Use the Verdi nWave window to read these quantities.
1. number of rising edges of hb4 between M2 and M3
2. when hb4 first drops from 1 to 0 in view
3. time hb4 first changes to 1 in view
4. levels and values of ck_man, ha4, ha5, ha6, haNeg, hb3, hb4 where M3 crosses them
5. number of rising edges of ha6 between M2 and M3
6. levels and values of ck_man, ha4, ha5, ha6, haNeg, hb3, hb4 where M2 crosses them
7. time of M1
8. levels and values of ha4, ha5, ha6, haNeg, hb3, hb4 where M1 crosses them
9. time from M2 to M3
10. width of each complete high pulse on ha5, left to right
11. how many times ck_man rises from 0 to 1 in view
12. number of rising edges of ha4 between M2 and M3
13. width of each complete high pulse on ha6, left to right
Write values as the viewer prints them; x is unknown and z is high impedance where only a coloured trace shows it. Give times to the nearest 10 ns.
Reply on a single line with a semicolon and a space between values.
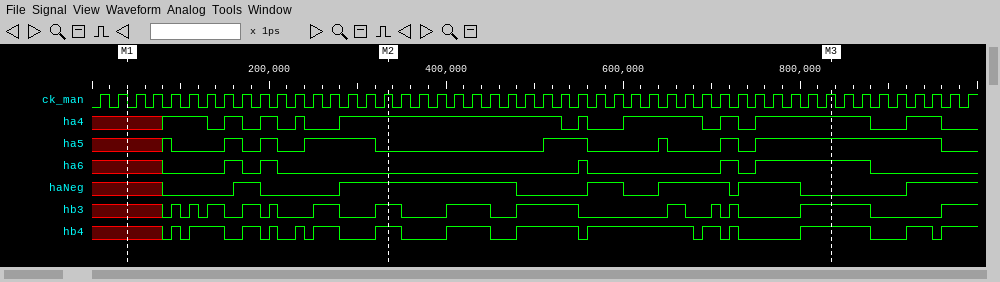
6; 100 ns; 90 ns; ck_man=1, ha4=1, ha5=1, ha6=1, haNeg=0, hb3=1, hb4=1; 3; ck_man=1, ha4=1, ha5=0, ha6=0, haNeg=1, hb3=1, hb4=1; 40 ns; ha4=x, ha5=x, ha6=x, haNeg=x, hb3=x, hb4=x; 500 ns; 20 ns, 20 ns, 80 ns, 50 ns, 10 ns, 20 ns, 210 ns; 50; 4; 20 ns, 20 ns, 10 ns, 20 ns, 130 ns
